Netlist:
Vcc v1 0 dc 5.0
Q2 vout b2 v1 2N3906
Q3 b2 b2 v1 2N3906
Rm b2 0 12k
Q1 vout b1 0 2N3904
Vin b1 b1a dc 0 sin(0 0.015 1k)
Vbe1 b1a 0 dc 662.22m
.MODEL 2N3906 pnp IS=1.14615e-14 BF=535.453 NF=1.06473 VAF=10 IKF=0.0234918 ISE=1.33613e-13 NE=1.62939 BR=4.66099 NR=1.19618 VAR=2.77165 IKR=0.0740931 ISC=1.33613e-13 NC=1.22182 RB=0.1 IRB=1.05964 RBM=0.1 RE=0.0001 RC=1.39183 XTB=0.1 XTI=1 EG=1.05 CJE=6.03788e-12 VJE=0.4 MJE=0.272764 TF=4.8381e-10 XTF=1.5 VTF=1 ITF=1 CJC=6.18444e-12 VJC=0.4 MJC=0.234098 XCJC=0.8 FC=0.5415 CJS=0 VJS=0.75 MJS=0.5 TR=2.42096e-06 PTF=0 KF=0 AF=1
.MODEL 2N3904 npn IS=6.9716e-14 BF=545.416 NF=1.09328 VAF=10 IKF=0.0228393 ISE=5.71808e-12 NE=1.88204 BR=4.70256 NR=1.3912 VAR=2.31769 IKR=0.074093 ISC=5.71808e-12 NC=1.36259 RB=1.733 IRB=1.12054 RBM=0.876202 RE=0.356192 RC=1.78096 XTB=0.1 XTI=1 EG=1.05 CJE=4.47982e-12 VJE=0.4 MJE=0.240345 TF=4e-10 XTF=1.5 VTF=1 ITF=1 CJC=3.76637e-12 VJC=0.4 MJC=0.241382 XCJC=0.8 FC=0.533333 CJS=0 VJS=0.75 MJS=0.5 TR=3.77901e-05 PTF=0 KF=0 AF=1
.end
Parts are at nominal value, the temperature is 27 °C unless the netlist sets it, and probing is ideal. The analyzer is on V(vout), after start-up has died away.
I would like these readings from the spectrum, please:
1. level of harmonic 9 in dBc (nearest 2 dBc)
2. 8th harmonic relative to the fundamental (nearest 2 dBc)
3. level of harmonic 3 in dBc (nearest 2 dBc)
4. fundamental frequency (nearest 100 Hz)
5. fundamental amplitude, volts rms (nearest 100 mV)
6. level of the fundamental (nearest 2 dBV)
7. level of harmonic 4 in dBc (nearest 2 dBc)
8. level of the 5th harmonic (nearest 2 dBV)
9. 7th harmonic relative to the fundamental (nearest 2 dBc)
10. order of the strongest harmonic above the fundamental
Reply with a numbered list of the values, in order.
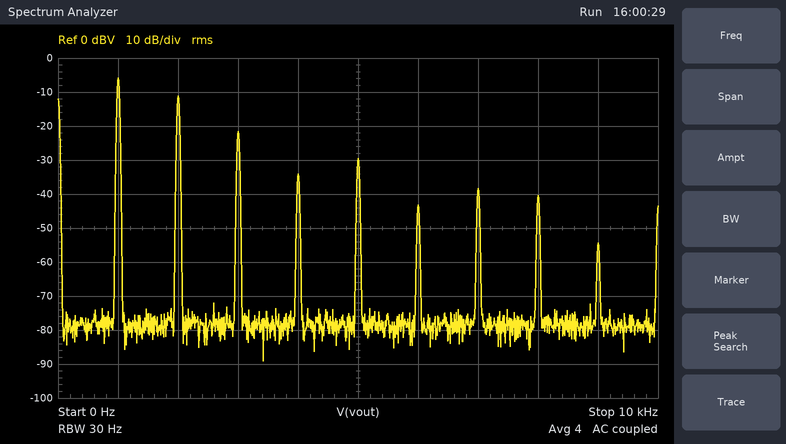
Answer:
1. -48 dBc
2. -34 dBc
3. -16 dBc
4. 1.0 kHz
5. 500 mV
6. -6 dBV
7. -28 dBc
8. -30 dBV
9. -32 dBc
10. 2
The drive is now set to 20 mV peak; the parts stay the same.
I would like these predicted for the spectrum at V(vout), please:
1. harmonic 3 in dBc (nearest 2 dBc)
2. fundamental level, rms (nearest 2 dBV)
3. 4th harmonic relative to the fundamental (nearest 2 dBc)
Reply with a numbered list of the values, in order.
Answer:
1. -18 dBc
2. -2 dBV
3. -24 dBc
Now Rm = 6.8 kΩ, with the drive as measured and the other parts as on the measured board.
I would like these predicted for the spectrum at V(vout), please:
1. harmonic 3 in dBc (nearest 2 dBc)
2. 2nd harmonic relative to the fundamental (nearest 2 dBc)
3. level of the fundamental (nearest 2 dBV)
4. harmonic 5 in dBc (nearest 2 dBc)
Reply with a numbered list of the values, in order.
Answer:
1. -30 dBc
2. -26 dBc
3. 4 dBV
4. -38 dBc
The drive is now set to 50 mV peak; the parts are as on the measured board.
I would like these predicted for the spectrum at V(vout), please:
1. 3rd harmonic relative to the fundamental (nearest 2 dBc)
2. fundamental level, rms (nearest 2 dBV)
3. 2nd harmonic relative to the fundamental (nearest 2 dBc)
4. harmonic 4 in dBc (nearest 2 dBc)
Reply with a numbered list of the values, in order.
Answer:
1. -22 dBc
2. 6 dBV
3. -8 dBc
4. -14 dBc
